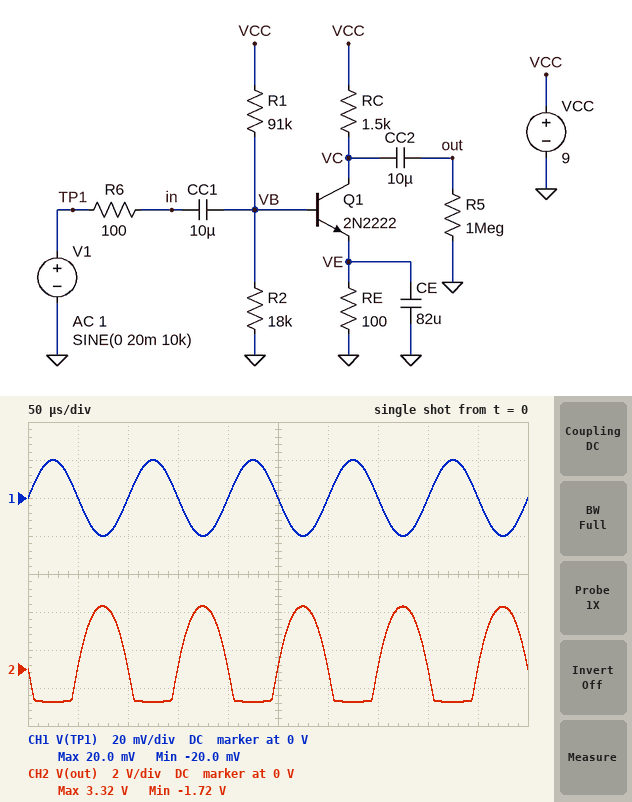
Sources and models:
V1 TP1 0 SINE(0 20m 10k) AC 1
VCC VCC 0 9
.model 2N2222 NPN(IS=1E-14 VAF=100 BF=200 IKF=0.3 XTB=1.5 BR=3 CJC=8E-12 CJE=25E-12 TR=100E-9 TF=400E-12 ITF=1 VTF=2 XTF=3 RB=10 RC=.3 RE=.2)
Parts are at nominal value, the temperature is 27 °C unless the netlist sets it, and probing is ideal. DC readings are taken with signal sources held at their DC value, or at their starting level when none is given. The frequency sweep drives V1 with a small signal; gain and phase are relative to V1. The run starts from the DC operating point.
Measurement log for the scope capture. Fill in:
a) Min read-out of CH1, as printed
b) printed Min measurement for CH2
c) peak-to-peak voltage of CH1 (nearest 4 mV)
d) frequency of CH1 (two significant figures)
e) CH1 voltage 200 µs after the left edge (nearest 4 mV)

-20.0 mV
-1.72 V
40 mV
10 kHz
0 V
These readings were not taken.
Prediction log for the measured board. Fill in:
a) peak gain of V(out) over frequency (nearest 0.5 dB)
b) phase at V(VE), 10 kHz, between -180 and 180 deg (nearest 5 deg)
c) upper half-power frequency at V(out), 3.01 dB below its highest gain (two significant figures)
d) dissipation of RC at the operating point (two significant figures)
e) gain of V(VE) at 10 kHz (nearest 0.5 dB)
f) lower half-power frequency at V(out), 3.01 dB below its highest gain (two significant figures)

46.5 dB
-90 deg
1.0 MHz
30 mW
-31.0 dB
310 Hz
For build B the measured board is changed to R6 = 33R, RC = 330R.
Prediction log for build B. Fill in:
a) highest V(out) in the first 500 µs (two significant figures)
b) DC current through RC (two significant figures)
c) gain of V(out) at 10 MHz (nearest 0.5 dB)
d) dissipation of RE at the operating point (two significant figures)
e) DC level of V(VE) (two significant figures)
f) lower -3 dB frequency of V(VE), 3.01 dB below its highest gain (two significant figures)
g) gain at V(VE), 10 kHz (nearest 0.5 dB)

830 mV
4.6 mA
32.0 dB
2.1 mW
460 mV
1.7 Hz
-30.0 dB
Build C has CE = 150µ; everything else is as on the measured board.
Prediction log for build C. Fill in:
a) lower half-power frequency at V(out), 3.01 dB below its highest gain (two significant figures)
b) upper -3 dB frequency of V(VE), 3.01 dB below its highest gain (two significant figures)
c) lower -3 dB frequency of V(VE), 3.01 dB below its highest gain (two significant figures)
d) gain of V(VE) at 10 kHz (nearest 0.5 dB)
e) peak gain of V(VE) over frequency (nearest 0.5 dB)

170 Hz
180 Hz
1.7 Hz
-36.5 dB
-1.5 dB
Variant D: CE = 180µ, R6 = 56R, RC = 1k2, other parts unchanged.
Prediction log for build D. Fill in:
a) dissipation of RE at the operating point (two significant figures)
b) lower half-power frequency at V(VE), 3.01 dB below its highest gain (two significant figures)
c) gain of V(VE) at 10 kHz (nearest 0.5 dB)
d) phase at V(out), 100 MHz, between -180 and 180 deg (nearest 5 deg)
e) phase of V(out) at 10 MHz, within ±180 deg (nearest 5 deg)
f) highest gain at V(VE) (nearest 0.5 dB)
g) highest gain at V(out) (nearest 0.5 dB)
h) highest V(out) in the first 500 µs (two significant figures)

2.1 mW
1.7 Hz
-37.5 dB
70 deg
100 deg
-1.5 dB
45.0 dB
2.8 V
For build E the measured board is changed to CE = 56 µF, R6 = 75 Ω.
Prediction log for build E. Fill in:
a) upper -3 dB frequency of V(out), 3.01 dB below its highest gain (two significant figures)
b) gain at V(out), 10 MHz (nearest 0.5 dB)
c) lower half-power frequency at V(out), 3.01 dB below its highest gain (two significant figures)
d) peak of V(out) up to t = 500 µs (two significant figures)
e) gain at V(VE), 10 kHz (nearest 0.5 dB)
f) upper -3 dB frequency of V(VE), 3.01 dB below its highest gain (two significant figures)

1.3 MHz
28.5 dB
450 Hz
3.4 V
-27.5 dB
460 Hz
